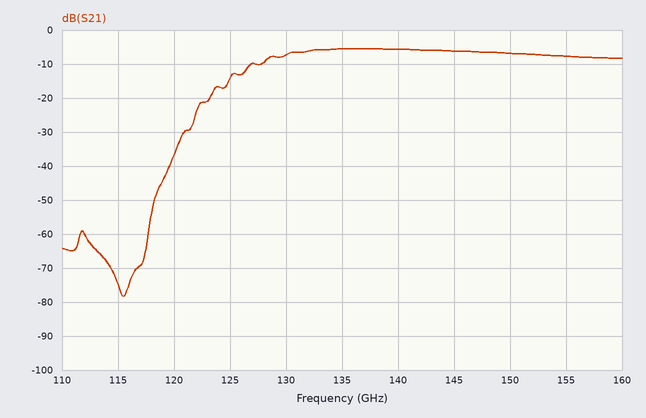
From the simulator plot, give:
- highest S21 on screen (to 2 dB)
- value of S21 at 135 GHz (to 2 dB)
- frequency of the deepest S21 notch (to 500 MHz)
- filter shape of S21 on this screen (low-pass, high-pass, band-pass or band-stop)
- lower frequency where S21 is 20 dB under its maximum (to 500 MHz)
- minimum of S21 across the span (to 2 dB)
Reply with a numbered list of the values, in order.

1. -6 dB
2. -6 dB
3. 115.5 GHz
4. high-pass
5. 122.0 GHz
6. -78 dB
